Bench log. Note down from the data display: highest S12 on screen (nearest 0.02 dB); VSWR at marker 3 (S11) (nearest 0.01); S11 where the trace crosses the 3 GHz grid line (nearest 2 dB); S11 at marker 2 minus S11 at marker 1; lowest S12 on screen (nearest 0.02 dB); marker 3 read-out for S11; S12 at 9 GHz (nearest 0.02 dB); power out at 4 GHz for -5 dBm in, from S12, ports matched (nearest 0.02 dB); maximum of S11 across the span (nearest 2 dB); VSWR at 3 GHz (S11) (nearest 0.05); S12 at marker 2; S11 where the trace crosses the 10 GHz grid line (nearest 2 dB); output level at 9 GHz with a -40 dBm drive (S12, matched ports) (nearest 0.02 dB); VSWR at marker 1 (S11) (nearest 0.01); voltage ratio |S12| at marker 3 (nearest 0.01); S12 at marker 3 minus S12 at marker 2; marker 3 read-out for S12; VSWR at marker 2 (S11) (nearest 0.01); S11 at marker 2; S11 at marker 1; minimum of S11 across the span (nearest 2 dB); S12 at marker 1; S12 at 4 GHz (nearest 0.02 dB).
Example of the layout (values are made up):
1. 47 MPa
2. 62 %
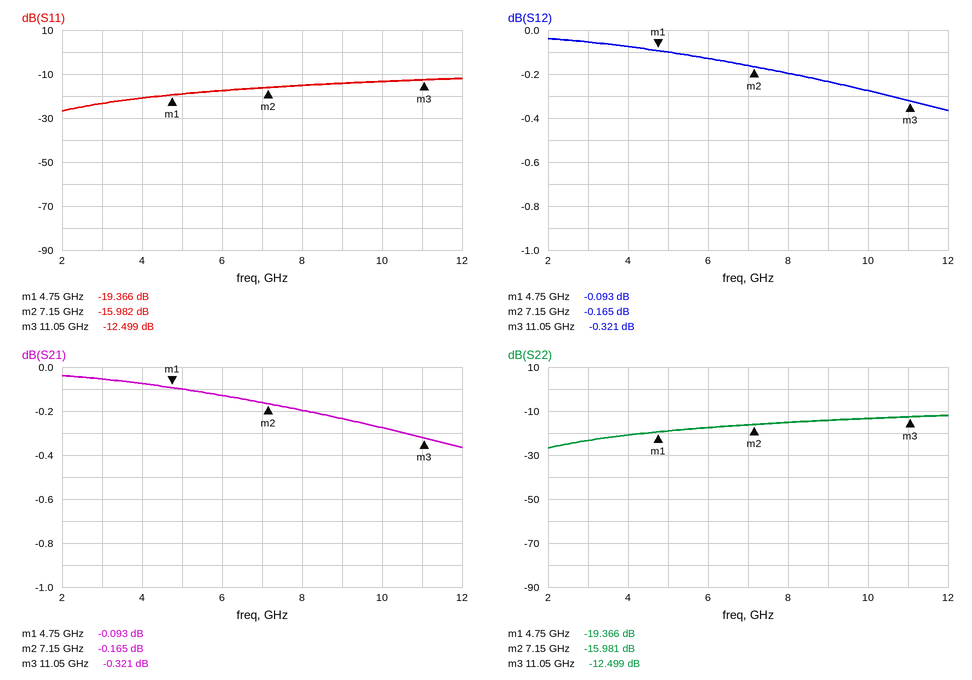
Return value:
1. -0.04 dB
2. 1.62
3. -24 dB
4. 3.384 dB
5. -0.36 dB
6. -12.499 dB
7. -0.24 dB
8. -5.08 dBm
9. -12 dB
10. 1.15
11. -0.165 dB
12. -14 dB
13. -40.24 dBm
14. 1.24
15. 0.96
16. -0.156 dB
17. -0.321 dB
18. 1.38
19. -15.982 dB
20. -19.366 dB
21. -26 dB
22. -0.093 dB
23. -0.08 dB
